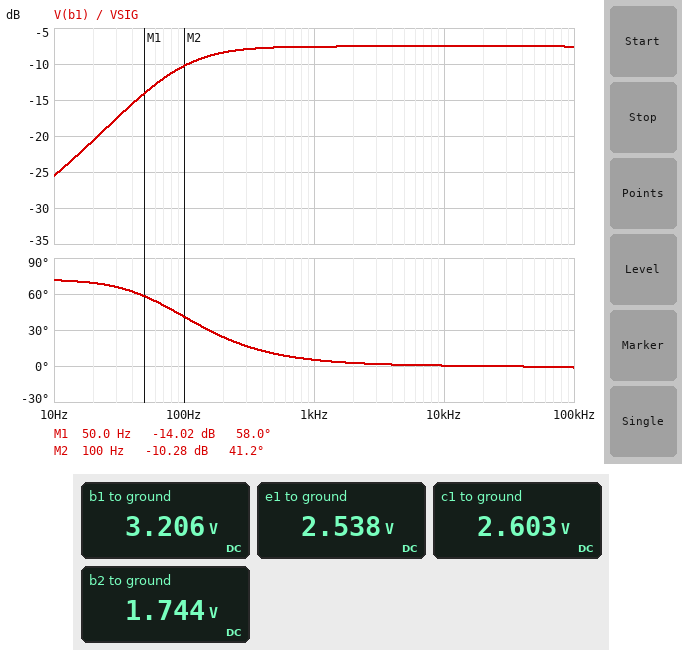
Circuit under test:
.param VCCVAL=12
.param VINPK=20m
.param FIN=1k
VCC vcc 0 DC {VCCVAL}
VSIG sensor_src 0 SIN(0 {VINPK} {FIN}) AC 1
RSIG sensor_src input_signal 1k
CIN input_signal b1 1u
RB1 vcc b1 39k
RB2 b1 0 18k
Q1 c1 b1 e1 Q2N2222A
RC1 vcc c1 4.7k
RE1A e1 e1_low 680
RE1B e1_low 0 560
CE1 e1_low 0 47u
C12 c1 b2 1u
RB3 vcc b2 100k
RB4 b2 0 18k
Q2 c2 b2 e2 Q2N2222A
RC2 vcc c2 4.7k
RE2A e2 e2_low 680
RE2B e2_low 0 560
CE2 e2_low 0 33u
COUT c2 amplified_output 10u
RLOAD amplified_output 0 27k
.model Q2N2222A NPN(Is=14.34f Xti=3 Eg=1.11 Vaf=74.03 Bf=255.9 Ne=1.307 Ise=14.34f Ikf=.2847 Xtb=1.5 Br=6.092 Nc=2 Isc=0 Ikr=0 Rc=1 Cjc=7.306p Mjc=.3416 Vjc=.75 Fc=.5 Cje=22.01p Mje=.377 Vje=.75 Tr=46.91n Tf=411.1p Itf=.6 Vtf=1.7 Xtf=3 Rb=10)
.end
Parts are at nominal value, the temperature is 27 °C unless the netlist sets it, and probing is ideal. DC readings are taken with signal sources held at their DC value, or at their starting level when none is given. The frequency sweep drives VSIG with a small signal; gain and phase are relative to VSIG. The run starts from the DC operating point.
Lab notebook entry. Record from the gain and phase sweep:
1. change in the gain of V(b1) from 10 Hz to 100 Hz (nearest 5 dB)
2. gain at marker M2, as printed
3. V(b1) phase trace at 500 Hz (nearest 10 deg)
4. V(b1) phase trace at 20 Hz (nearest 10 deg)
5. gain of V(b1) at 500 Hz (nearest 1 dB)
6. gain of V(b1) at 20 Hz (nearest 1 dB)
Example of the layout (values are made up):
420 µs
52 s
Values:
15 dB
-10.28 dB
10 deg
70 deg
-8 dB
-21 dB
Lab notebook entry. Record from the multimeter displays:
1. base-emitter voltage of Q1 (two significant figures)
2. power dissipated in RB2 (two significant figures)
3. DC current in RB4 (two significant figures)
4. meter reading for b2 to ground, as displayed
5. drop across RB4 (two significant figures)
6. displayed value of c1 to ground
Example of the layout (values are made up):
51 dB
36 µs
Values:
670 mV
570 µW
97 µA
1.744 V
1.7 V
2.603 V
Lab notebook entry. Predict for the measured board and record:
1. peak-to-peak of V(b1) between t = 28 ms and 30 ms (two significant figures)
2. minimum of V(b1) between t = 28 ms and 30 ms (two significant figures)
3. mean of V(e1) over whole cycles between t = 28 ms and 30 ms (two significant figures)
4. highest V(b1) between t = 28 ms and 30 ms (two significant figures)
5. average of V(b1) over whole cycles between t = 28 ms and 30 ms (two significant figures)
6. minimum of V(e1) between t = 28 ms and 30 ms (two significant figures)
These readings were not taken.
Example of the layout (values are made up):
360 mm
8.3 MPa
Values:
17 mV
3.2 V
2.5 V
3.2 V
3.2 V
2.5 V
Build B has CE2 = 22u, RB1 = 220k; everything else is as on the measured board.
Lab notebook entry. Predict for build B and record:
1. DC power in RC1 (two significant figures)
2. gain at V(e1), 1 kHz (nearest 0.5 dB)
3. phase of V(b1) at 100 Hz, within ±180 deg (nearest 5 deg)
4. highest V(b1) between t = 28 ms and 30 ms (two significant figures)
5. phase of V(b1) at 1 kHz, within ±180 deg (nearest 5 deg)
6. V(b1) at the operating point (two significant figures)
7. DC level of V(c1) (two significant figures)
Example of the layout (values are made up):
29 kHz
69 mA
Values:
230 µW
-2.0 dB
5 deg
900 mV
0 deg
880 mV
11 V
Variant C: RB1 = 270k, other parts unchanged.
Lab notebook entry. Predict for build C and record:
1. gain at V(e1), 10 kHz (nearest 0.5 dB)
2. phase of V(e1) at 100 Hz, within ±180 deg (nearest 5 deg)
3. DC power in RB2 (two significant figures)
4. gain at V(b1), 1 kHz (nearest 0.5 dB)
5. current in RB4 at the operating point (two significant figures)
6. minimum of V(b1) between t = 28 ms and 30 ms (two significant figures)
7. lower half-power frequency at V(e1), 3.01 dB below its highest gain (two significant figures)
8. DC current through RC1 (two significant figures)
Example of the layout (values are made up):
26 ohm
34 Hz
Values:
-3.0 dB
5 deg
30 µW
-0.5 dB
97 µA
720 mV
8.7 Hz
120 µA
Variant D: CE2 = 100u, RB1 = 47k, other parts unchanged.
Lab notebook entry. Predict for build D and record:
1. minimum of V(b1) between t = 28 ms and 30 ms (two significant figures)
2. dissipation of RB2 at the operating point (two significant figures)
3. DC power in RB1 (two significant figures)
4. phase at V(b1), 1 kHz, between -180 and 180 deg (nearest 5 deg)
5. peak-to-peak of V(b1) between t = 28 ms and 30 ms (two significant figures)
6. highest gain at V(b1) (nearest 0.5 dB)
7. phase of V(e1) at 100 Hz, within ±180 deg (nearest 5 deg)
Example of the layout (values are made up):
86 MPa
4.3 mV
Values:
3.1 V
550 µW
1.7 mW
0 deg
33 mV
-2.0 dB
15 deg
